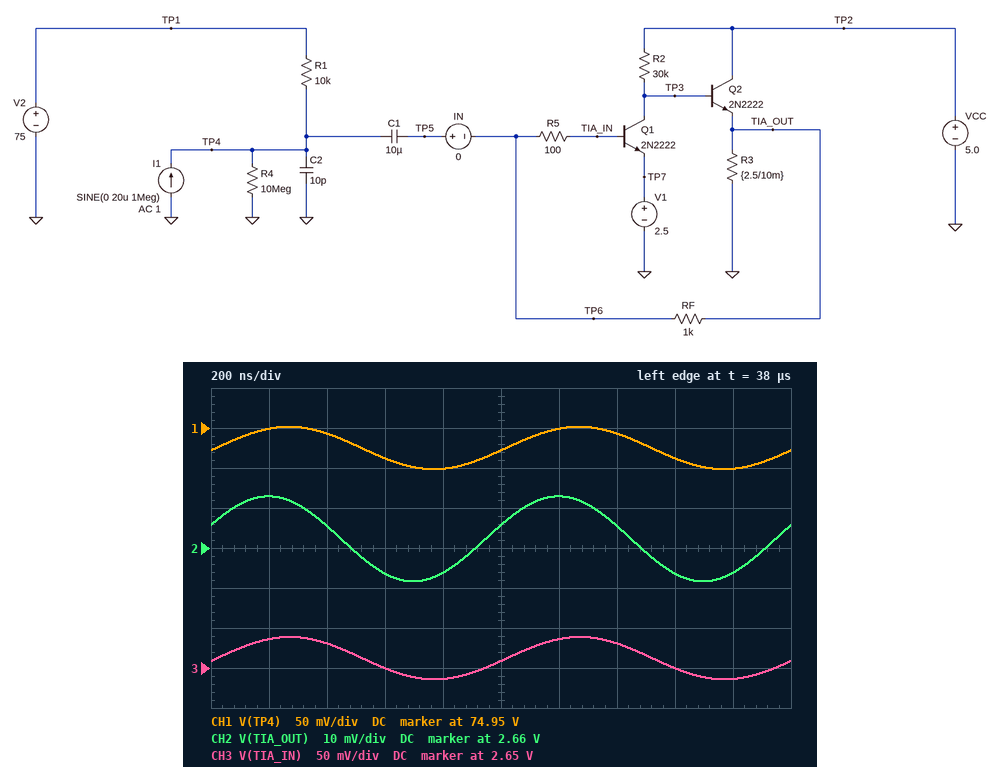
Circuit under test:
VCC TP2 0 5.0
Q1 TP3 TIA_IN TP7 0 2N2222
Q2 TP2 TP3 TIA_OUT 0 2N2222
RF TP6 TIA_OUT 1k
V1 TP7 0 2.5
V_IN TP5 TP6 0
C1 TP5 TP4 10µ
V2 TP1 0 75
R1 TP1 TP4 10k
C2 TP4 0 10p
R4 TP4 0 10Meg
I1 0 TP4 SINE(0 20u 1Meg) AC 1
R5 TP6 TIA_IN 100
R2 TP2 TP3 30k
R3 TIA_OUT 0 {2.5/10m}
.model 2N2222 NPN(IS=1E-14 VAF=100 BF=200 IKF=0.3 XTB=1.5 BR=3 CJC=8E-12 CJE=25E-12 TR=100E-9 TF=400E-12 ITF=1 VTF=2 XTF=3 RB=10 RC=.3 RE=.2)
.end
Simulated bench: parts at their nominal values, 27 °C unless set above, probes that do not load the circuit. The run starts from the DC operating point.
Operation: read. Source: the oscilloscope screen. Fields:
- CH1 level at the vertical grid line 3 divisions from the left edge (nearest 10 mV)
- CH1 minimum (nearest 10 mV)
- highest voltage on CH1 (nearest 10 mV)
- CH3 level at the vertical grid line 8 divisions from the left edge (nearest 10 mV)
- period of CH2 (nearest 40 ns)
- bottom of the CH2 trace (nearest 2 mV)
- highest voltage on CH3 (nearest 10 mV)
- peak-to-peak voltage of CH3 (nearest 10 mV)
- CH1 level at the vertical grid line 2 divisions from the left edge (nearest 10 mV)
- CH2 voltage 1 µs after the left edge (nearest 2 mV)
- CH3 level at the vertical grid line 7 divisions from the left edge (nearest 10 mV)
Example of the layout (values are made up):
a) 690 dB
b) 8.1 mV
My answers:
a) 74.91 V
b) 74.90 V
c) 74.95 V
d) 2.65 V
e) 1.00 µs
f) 2.652 V
g) 2.69 V
h) 50 mV
i) 74.94 V
j) 2.666 V
k) 2.68 V
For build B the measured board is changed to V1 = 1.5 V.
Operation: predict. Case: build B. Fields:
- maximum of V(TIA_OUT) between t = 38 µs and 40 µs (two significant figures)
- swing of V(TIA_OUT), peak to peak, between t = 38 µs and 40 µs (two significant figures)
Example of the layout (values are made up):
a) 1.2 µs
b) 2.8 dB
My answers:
a) 2.1 V
b) 39 mV
